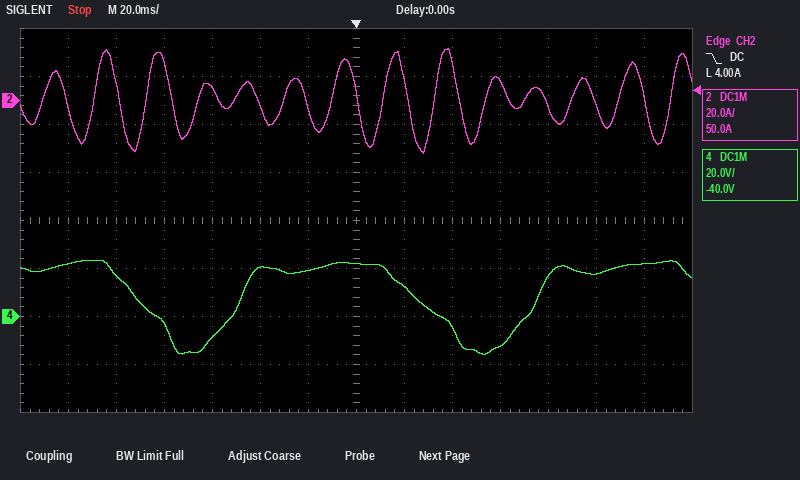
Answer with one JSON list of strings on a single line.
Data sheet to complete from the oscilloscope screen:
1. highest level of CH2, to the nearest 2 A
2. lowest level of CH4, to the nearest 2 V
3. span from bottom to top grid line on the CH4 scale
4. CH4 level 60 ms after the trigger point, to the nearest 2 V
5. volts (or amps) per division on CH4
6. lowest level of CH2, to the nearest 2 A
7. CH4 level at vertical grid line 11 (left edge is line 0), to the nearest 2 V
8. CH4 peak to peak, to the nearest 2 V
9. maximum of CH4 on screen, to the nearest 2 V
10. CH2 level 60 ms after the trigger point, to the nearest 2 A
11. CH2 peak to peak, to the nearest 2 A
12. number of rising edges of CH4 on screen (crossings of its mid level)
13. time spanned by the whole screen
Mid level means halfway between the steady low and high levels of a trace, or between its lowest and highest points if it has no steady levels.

["22 A", "-16 V", "160 V", "-12 V", "20 V", "-22 A", "16 V", "40 V", "24 V", "8 A", "44 A", "2", "280 ms"]
